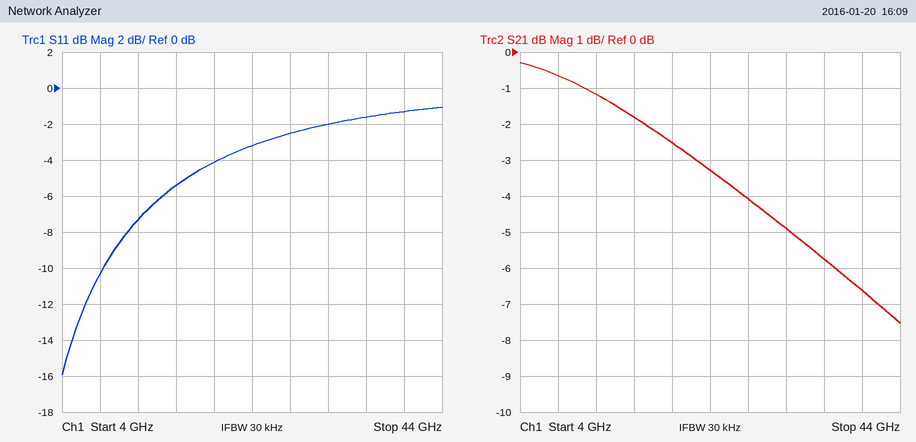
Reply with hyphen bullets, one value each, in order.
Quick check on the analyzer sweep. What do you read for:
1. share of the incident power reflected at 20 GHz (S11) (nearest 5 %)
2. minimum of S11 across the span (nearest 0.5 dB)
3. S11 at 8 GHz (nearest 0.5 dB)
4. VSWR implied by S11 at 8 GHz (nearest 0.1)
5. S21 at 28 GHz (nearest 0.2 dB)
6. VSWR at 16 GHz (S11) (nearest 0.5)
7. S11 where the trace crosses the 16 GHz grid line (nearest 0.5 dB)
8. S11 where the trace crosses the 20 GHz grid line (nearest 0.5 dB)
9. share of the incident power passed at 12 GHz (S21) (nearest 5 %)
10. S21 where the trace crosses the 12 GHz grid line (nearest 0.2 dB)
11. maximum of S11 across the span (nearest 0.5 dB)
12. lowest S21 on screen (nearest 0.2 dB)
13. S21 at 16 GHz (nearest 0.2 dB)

- 40 %
- -16.0 dB
- -10.5 dB
- 1.9
- -4.0 dB
- 3.5
- -5.5 dB
- -4.0 dB
- 75 %
- -1.2 dB
- -1.0 dB
- -7.6 dB
- -1.8 dB
